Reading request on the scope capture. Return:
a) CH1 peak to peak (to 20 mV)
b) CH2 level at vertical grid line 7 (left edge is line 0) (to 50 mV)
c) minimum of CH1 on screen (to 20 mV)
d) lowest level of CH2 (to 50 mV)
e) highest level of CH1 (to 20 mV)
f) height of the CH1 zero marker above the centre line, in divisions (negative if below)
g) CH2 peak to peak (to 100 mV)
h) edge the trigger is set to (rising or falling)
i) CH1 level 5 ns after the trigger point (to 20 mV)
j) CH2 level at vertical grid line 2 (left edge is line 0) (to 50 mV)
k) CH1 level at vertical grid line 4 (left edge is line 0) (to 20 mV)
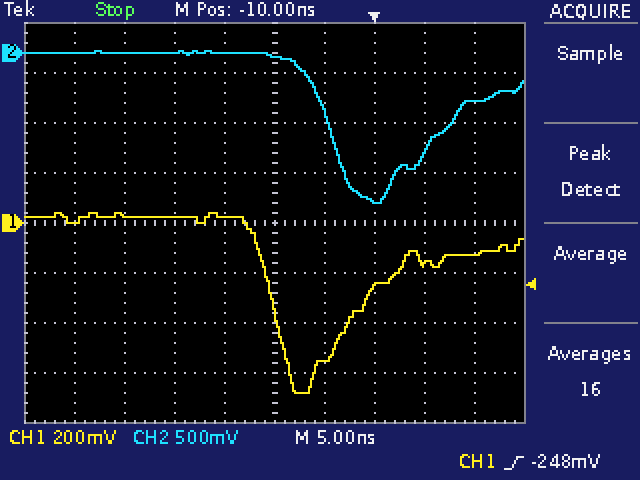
720 mV
-1.50 V
-680 mV
-1.50 V
40 mV
0.0 div
1.50 V
rising
-160 mV
0 mV
20 mV
